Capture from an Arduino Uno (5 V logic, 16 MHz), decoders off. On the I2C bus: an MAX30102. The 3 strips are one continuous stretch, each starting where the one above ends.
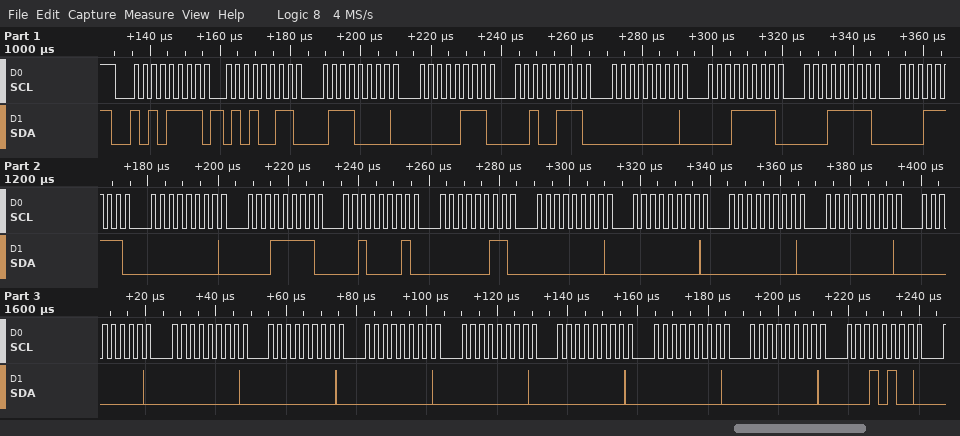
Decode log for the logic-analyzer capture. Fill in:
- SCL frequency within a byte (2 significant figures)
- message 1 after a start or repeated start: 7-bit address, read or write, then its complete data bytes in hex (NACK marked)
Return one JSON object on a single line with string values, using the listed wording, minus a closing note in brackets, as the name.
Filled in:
{"SCL frequency within a byte": "400 kHz", "message 1 after a start or repeated start: 7-bit address, read or write, then its complete data bytes in hex": "0x57 read: 53 70 07 27 00 1F 1F 1F 00 1F 21 03 00 00 00 00 00 00 00 00 00 00 00 00 14"}
